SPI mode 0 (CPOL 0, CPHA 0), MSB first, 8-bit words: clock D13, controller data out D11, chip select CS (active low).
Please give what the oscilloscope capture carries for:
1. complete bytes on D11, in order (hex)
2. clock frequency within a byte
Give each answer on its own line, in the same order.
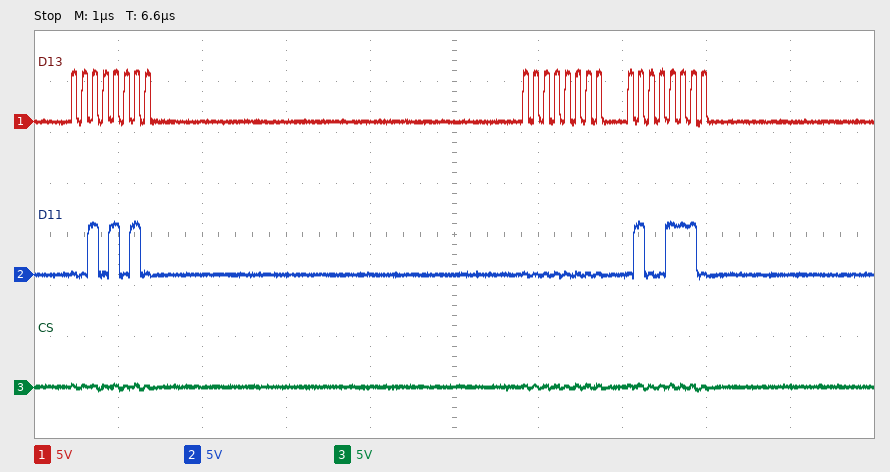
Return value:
2A 00 4E
8 MHz
